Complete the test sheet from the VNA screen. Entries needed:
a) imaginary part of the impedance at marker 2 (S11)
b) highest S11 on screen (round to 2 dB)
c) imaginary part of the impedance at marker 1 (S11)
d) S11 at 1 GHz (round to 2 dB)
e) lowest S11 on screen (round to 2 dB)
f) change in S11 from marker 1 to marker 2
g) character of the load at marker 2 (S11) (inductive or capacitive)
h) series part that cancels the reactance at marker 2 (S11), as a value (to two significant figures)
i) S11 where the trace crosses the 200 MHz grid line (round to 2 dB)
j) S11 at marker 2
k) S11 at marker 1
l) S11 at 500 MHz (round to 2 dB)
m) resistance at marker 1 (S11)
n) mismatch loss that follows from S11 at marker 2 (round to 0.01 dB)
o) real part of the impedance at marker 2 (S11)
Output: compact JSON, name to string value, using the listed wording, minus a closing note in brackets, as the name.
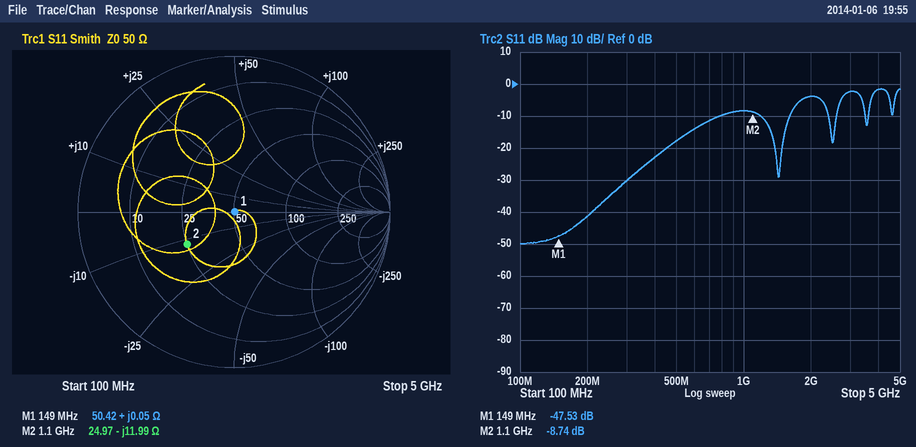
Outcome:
{"imaginary part of the impedance at marker 2": "-11.99 Ω", "highest S11 on screen": "-2 dB", "imaginary part of the impedance at marker 1": "+0.05 Ω", "S11 at 1 GHz": "-8 dB", "lowest S11 on screen": "-50 dB", "change in S11 from marker 1 to marker 2": "38.79 dB", "character of the load at marker 2 (S11)": "capacitive", "series part that cancels the reactance at marker 2 (S11), as a value": "1.7 nH", "S11 where the trace crosses the 200 MHz grid line": "-42 dB", "S11 at marker 2": "-8.74 dB", "S11 at marker 1": "-47.53 dB", "S11 at 500 MHz": "-18 dB", "resistance at marker 1": "50.42 Ω", "mismatch loss that follows from S11 at marker 2": "0.62 dB", "real part of the impedance at marker 2": "24.97 Ω"}
